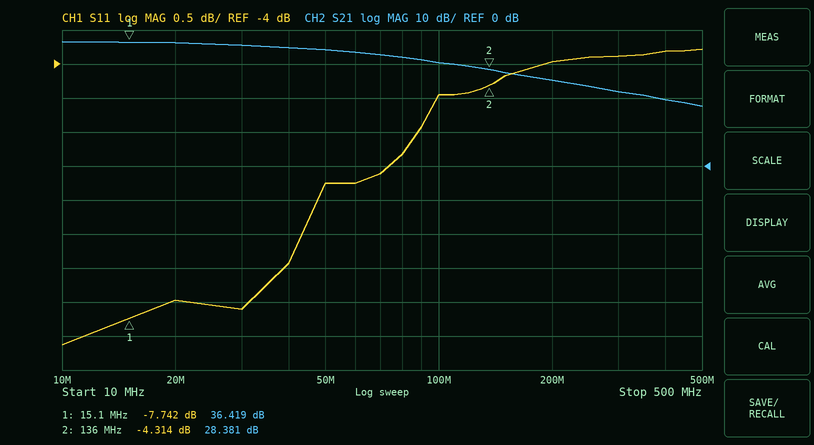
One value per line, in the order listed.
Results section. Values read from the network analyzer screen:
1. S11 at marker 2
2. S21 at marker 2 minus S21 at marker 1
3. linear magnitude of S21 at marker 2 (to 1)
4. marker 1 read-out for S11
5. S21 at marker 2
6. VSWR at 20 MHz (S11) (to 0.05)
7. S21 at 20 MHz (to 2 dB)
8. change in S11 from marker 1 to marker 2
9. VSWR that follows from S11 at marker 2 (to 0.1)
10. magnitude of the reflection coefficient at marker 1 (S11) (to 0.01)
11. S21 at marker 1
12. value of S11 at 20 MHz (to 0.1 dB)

-4.314 dB
-8.038 dB
26
-7.742 dB
28.381 dB
2.45
36 dB
3.428 dB
4.1
0.41
36.419 dB
-7.5 dB
